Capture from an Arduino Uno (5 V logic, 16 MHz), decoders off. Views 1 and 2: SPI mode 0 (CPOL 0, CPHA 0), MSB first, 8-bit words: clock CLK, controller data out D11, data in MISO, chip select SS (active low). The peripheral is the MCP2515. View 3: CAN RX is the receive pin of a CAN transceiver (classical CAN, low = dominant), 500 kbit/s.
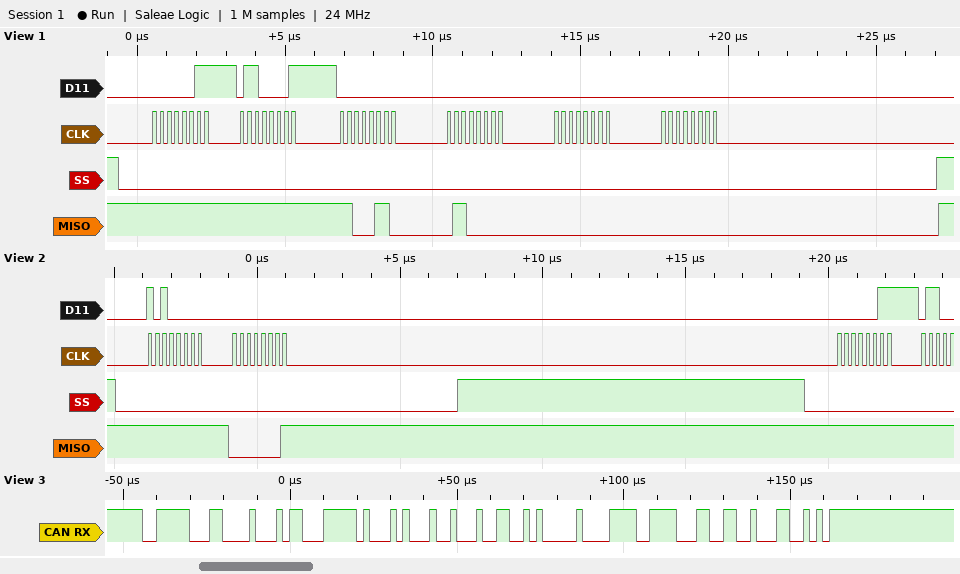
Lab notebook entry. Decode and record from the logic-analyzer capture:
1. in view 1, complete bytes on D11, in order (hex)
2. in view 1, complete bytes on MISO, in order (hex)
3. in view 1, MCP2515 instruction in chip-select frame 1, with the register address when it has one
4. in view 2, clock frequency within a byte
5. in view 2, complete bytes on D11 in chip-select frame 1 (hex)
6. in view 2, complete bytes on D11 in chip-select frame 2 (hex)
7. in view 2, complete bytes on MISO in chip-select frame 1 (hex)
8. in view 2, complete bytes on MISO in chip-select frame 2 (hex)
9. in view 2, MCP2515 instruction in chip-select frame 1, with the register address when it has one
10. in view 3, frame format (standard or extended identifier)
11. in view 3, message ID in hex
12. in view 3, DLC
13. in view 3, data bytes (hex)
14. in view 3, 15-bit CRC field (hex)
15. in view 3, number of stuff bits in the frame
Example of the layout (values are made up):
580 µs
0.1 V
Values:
0x03 0x61 0x00 0x00 0x00 0x00
0xFF 0xFF 0xC6 0x60 0x00 0x00
READ 0x61
4 MHz
A0 00
03
FF 01
FF
READ STATUS
standard
0x3E6
8
B1 F8 A2 44 CA 00 F3 C6
0x3232
3
